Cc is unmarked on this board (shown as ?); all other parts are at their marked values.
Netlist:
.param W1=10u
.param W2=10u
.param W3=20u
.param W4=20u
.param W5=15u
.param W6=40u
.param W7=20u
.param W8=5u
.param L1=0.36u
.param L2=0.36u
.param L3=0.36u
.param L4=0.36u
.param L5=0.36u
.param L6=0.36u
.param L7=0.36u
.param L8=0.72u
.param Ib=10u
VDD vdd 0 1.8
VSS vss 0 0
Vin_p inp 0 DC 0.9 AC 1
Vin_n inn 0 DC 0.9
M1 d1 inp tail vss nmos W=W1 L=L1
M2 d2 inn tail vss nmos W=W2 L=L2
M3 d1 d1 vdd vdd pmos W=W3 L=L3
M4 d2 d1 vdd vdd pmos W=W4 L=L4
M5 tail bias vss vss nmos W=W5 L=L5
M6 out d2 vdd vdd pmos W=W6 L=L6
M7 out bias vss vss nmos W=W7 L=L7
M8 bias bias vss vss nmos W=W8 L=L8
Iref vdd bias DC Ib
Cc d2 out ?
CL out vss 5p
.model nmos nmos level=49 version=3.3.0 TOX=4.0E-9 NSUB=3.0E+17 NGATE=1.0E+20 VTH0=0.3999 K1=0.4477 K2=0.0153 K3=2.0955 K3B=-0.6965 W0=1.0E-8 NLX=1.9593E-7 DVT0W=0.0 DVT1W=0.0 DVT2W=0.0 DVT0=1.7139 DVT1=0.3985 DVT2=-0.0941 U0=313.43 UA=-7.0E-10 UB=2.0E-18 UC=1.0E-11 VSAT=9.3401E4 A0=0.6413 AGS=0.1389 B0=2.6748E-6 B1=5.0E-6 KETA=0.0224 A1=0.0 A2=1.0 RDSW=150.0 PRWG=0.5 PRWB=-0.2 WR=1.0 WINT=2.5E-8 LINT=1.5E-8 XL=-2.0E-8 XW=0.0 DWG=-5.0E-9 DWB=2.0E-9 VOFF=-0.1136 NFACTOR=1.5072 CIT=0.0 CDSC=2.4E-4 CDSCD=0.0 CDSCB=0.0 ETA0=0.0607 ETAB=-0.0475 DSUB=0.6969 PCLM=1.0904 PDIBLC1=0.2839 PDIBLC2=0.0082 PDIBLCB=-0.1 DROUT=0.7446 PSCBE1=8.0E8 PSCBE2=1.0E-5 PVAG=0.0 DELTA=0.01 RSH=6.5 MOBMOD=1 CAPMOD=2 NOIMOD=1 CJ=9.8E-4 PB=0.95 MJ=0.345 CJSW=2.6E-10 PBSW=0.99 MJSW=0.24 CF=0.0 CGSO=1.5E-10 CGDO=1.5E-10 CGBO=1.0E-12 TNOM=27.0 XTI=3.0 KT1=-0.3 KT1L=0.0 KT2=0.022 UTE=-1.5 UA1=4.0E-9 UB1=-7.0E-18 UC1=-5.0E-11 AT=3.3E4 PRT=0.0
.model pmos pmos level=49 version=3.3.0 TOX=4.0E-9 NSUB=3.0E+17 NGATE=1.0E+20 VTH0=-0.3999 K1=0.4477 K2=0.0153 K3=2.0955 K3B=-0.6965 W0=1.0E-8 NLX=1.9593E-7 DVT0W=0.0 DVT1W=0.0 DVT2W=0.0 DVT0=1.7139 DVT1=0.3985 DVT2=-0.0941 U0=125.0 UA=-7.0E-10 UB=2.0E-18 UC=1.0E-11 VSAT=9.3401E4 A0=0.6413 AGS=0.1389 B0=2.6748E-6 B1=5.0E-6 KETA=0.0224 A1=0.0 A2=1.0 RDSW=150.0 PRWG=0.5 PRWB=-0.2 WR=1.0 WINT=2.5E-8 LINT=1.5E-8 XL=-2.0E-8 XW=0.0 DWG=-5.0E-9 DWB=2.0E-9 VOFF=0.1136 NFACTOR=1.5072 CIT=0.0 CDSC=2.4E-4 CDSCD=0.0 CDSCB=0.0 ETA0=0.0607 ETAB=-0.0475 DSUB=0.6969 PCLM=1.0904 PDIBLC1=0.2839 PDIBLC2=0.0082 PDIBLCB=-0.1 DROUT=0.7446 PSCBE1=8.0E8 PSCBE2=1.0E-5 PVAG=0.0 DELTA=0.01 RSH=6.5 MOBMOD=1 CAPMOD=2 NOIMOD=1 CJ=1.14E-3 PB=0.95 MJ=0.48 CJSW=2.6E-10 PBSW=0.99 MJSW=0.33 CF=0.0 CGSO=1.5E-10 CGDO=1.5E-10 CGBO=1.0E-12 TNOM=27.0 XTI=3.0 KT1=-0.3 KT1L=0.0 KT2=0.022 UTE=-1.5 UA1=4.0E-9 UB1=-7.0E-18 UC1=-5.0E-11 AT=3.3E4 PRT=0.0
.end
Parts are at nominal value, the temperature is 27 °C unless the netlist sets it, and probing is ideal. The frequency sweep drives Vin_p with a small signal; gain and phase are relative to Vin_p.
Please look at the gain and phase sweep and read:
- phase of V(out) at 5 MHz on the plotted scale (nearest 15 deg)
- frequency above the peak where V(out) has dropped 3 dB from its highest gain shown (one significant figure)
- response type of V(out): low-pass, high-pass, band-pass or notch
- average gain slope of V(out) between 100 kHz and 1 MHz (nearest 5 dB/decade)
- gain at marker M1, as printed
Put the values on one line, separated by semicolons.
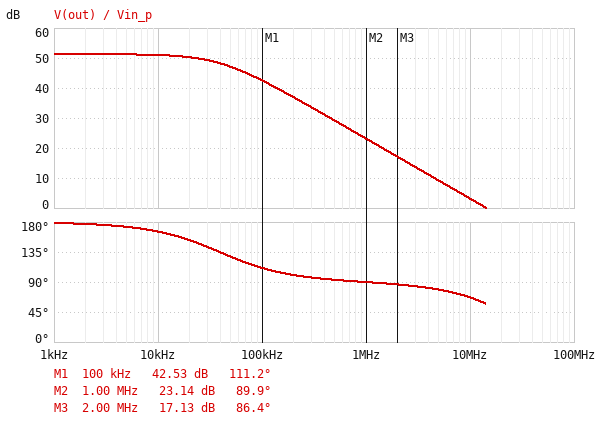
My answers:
75 deg; 40 kHz; low-pass; -20 dB/decade; 42.53 dB
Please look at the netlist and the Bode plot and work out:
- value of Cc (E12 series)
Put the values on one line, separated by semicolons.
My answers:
4.7 pF
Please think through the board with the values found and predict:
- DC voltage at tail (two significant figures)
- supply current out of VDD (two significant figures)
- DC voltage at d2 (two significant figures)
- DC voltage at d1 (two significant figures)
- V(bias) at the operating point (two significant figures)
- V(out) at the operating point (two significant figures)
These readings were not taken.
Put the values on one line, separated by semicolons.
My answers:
320 mV; 130 µA; 1.0 V; 1.0 V; 540 mV; 110 mV
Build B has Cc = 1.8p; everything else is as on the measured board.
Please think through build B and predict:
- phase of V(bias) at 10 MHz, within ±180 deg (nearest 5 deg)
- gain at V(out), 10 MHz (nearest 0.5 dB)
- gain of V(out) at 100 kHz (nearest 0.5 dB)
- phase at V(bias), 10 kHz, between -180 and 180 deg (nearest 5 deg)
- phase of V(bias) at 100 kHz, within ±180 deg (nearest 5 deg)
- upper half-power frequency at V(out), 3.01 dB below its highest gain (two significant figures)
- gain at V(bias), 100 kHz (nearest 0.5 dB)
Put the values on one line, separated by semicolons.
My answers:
160 deg; 11.0 dB; 48.5 dB; -95 deg; -135 deg; 100 kHz; -48.0 dB
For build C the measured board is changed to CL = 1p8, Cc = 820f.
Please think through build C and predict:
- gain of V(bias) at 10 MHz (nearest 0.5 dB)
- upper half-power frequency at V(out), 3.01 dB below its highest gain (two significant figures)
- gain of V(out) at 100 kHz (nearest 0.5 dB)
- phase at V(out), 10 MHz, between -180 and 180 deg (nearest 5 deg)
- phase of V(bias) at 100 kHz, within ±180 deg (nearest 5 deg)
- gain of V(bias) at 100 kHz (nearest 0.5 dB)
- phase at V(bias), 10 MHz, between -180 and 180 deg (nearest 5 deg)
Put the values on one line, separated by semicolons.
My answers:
-38.0 dB; 220 kHz; 50.5 dB; 85 deg; -115 deg; -45.5 dB; 170 deg
